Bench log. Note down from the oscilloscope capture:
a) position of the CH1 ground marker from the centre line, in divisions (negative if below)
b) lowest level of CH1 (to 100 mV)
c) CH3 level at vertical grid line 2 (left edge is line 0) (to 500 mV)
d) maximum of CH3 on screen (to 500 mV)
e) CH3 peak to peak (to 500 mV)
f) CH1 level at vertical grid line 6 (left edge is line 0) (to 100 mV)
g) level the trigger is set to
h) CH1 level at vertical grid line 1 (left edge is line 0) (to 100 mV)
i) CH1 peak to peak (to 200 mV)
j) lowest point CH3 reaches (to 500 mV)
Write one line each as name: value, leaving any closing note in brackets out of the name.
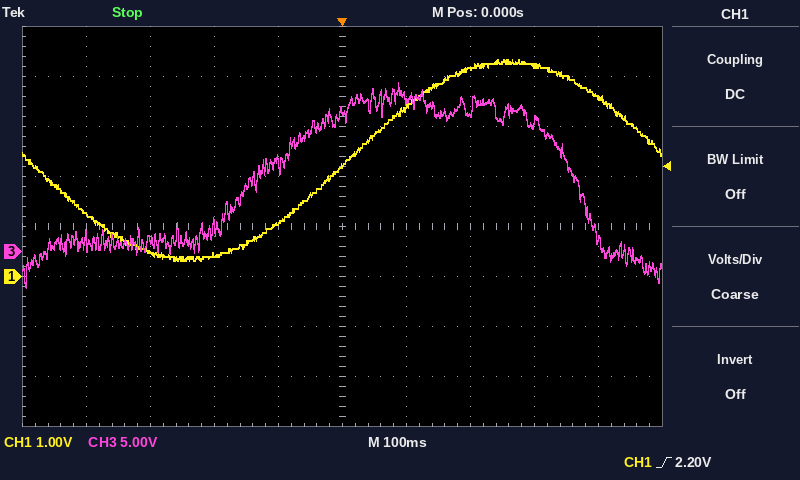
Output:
position of the CH1 ground marker from the centre line, in divisions: -1.0 div
lowest level of CH1: 300 mV
CH3 level at vertical grid line 2 (left edge is line 0): 1.0 V
maximum of CH3 on screen: 17.0 V
CH3 peak to peak: 20.5 V
CH1 level at vertical grid line 6 (left edge is line 0): 3.4 V
level the trigger is set to: 2.20 V
CH1 level at vertical grid line 1 (left edge is line 0): 1.3 V
CH1 peak to peak: 4.0 V
lowest point CH3 reaches: -3.5 V
